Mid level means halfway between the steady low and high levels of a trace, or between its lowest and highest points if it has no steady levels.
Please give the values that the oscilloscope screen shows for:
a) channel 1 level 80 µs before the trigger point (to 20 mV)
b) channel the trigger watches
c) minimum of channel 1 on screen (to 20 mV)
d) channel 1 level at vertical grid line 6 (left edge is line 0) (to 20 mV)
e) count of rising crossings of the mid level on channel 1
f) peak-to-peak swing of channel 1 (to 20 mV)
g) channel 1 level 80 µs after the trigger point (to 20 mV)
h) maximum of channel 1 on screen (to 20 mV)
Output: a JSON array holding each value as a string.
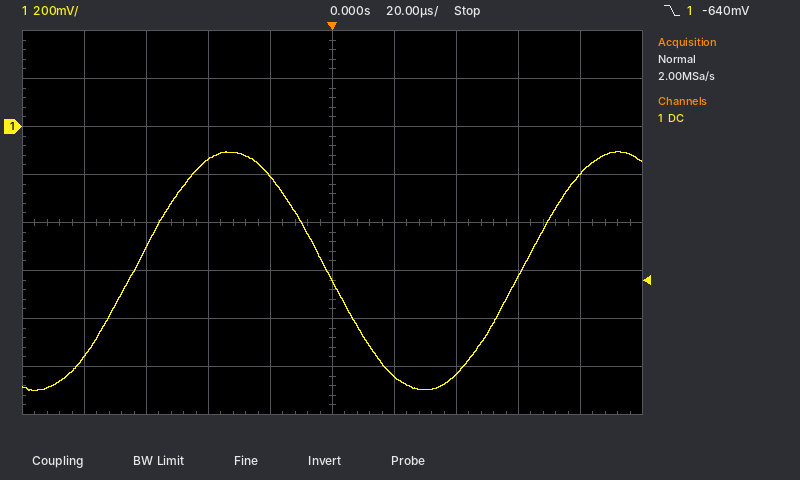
["-960 mV", "channel 1", "-1.10 V", "-1.04 V", "2", "1.00 V", "-200 mV", "-100 mV"]
